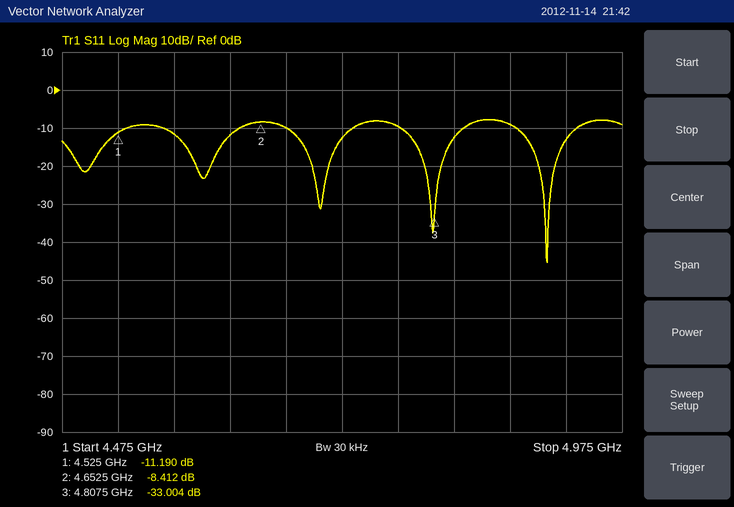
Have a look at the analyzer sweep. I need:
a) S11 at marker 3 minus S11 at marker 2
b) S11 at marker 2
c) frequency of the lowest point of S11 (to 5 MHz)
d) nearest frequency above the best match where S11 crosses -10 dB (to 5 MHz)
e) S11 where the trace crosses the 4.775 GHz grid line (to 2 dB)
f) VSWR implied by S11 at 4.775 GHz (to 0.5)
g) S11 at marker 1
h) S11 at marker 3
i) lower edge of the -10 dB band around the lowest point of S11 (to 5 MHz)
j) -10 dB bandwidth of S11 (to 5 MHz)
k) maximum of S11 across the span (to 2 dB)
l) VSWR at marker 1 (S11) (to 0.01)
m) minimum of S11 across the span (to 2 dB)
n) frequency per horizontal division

-24.592 dB
-8.412 dB
4.910 GHz
4.935 GHz
-10 dB
2.0
-11.190 dB
-33.004 dB
4.880 GHz
55 MHz
-8 dB
1.76
-46 dB
50 MHz
